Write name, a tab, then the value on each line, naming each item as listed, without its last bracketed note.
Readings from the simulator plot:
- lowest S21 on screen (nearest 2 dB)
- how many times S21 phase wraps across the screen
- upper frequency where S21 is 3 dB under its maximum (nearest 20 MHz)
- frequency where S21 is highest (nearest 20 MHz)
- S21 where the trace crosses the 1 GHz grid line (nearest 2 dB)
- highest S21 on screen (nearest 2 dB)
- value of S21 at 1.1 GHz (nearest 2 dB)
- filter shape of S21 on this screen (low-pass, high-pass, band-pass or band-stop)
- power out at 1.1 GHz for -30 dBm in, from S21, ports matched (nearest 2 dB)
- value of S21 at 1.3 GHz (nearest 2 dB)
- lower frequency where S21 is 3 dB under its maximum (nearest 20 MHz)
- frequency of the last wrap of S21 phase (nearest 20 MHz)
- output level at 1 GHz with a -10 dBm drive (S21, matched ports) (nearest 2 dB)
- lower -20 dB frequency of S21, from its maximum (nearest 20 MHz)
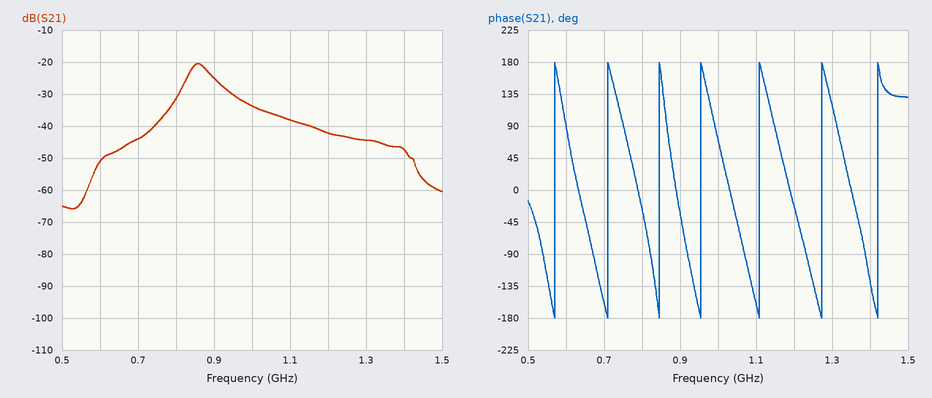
lowest S21 on screen	-66 dB
how many times S21 phase wraps across the screen	7
upper frequency where S21 is 3 dB under its maximum	880 MHz
frequency where S21 is highest	860 MHz
S21 where the trace crosses the 1 GHz grid line	-34 dB
highest S21 on screen	-20 dB
value of S21 at 1.1 GHz	-38 dB
filter shape of S21 on this screen	band-pass
power out at 1.1 GHz for -30 dBm in, from S21, ports matched	-68 dBm
value of S21 at 1.3 GHz	-44 dB
lower frequency where S21 is 3 dB under its maximum	840 MHz
frequency of the last wrap of S21 phase	1.42 GHz
output level at 1 GHz with a -10 dBm drive (S21, matched ports)	-44 dBm
lower -20 dB frequency of S21, from its maximum	740 MHz
